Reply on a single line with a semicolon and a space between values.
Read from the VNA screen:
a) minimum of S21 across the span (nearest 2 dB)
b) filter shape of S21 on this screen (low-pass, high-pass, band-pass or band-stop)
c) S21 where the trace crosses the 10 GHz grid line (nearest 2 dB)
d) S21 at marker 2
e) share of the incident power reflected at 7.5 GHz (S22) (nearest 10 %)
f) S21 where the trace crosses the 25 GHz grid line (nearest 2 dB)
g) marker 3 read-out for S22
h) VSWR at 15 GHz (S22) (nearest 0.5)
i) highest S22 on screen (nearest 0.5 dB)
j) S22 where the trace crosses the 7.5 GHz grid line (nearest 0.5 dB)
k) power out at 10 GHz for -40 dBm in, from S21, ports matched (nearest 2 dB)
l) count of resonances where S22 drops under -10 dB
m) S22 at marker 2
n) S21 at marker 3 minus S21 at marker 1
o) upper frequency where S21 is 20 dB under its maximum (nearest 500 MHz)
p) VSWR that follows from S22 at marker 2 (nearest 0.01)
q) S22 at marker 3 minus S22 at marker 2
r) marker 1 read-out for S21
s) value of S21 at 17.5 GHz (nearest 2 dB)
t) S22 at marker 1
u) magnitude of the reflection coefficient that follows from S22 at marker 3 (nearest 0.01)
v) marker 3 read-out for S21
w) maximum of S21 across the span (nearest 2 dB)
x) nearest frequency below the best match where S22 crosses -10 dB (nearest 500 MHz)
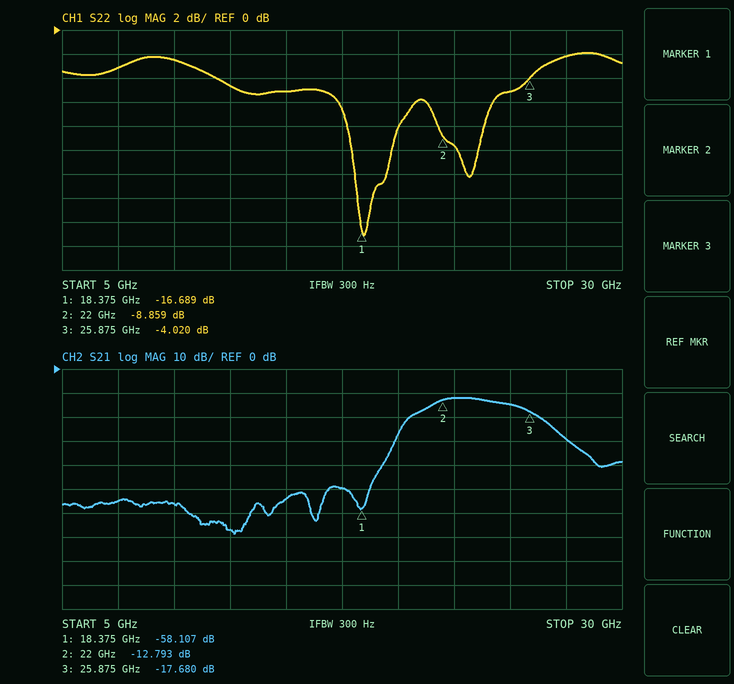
-68 dB; band-pass; -56 dB; -12.793 dB; 50 %; -14 dB; -4.020 dB; 3.5; -2.0 dB; -3.0 dB; -96 dBm; 2; -8.859 dB; 40.427 dB; 28.0 GHz; 2.13; 4.839 dB; -58.107 dB; -50 dB; -16.689 dB; 0.63; -17.680 dB; -12 dB; 18.0 GHz
